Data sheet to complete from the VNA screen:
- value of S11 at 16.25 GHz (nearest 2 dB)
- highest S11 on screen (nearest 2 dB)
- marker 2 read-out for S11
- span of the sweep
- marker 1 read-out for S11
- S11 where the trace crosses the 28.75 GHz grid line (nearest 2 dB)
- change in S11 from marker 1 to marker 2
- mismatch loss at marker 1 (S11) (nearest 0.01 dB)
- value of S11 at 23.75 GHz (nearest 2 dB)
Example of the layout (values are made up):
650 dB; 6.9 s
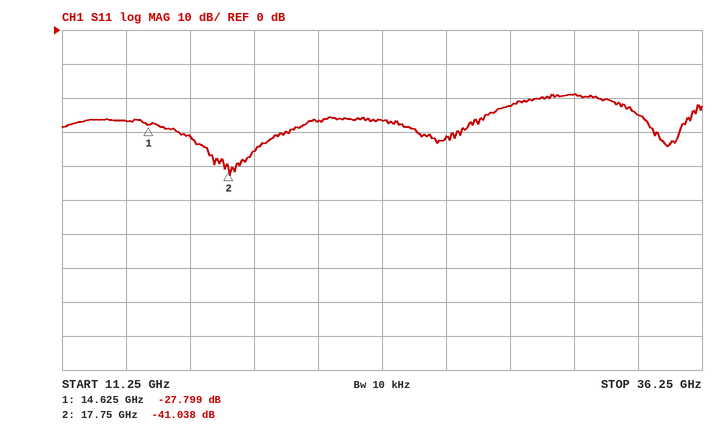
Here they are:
-32 dB; -18 dB; -41.038 dB; 25 GHz; -27.799 dB; -22 dB; -13.239 dB; 0.01 dB; -26 dB
